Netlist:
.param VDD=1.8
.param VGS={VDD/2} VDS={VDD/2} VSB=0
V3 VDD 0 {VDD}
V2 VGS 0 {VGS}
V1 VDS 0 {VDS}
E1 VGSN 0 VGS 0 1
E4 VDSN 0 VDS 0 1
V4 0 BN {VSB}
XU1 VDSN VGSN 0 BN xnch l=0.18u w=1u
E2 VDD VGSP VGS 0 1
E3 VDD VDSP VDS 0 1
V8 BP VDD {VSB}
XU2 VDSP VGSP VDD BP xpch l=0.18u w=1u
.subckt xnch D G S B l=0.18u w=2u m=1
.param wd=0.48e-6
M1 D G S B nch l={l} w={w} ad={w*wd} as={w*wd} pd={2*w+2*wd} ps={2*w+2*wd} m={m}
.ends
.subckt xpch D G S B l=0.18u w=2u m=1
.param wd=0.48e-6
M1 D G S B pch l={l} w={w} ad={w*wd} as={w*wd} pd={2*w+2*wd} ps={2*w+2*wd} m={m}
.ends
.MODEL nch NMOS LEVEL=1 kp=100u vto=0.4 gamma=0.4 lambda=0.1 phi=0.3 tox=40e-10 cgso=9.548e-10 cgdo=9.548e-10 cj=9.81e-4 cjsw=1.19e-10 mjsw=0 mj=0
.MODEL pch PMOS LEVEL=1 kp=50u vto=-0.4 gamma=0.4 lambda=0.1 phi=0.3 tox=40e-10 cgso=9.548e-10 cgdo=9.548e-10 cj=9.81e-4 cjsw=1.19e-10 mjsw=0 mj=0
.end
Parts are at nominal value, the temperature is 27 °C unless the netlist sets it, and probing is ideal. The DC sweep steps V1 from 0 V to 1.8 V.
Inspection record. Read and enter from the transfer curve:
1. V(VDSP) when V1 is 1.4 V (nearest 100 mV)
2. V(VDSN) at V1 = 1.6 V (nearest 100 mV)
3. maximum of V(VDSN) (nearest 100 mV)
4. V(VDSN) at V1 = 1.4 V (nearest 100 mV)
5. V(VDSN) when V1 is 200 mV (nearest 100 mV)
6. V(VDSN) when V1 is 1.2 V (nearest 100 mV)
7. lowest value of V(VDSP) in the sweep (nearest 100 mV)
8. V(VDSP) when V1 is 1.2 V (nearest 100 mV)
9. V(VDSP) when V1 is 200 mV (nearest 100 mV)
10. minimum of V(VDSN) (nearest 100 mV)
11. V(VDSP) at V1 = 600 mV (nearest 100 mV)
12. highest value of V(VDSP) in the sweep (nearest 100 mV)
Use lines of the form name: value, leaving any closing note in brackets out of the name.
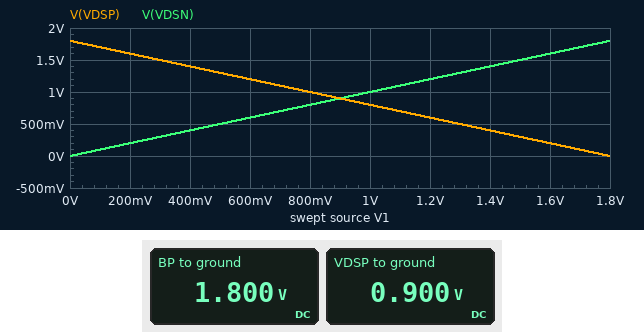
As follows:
V(VDSP) when V1 is 1.4 V: 400 mV
V(VDSN) at V1 = 1.6 V: 1.6 V
maximum of V(VDSN): 1.8 V
V(VDSN) at V1 = 1.4 V: 1.4 V
V(VDSN) when V1 is 200 mV: 200 mV
V(VDSN) when V1 is 1.2 V: 1.2 V
lowest value of V(VDSP) in the sweep: 0 V
V(VDSP) when V1 is 1.2 V: 600 mV
V(VDSP) when V1 is 200 mV: 1.6 V
minimum of V(VDSN): 0 V
V(VDSP) at V1 = 600 mV: 1.2 V
highest value of V(VDSP) in the sweep: 1.8 V
